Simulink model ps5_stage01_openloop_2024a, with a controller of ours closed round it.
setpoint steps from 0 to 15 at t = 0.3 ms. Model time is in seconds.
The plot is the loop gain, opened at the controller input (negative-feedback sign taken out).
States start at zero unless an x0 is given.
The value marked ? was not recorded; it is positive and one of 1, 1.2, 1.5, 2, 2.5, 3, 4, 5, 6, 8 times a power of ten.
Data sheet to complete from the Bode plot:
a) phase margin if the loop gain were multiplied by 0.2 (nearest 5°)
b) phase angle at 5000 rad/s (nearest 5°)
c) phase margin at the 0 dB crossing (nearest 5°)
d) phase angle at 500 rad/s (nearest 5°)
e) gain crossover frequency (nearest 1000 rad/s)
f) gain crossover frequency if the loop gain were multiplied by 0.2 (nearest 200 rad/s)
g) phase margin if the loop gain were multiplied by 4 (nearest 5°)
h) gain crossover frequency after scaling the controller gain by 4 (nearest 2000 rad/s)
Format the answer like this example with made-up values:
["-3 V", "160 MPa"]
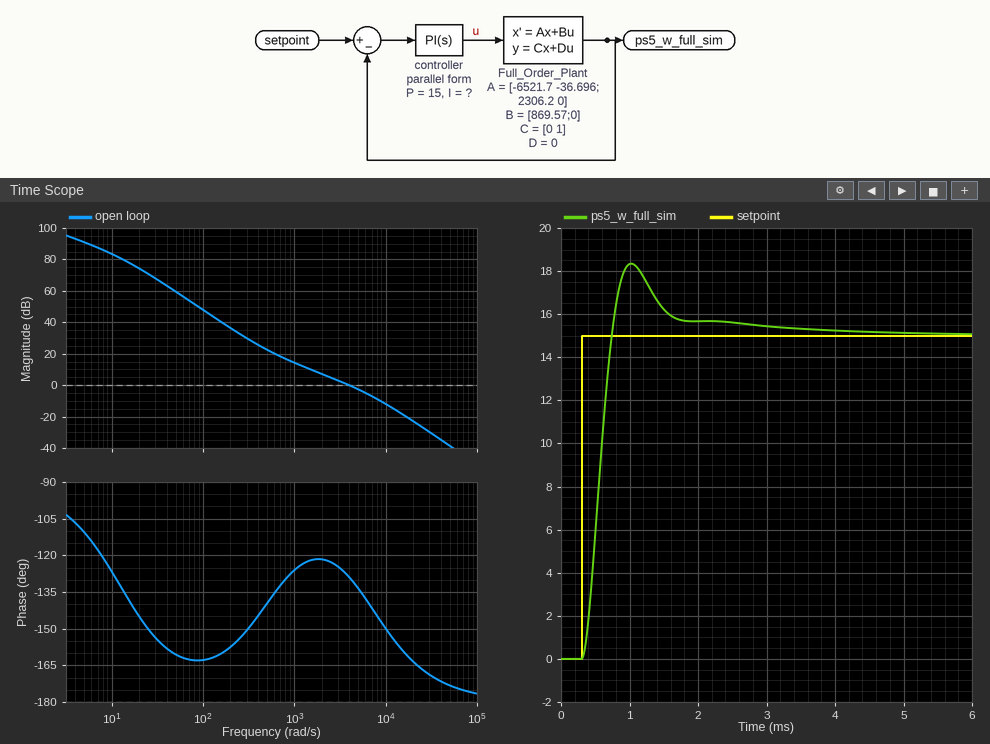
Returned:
["55°", "-135°", "50°", "-140°", "4000 rad/s", "1000 rad/s", "30°", "10000 rad/s"]
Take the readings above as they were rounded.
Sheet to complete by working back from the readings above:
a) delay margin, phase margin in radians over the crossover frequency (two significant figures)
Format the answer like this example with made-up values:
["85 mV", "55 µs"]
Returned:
["0.00022 s"]
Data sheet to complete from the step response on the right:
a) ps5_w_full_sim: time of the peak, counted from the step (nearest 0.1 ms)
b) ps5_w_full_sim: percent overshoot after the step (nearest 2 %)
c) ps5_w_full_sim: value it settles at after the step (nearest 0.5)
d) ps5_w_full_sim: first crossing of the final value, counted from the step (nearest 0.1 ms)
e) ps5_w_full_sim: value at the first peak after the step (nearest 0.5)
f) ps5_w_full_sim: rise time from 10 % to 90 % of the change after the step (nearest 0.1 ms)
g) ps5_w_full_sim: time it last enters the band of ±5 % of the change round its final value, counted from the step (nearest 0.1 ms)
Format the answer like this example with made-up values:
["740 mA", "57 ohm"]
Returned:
["0.7 ms", "22 %", "15.0", "0.4 ms", "18.5", "0.3 ms", "1.4 ms"]
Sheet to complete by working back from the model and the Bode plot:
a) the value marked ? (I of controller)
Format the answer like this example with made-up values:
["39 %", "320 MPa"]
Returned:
["8000"]
